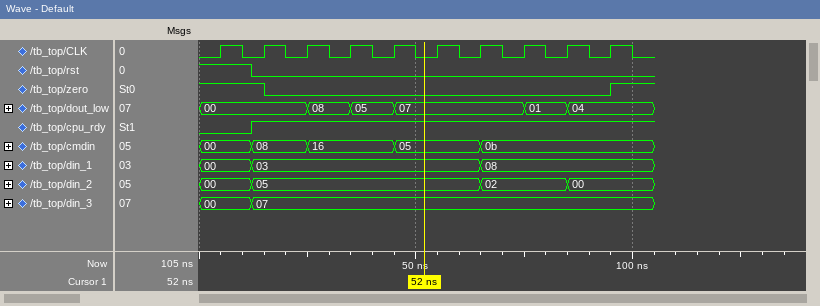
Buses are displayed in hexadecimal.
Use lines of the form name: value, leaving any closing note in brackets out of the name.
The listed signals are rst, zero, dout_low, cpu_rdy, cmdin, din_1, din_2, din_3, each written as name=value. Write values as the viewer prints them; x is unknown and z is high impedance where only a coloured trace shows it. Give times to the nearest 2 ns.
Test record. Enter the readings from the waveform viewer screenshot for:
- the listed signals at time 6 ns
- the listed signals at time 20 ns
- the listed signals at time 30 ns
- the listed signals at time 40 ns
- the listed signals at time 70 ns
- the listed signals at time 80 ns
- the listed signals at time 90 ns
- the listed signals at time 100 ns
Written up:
the listed signals at time 6 ns: rst=1, zero=1, dout_low=00, cpu_rdy=0, cmdin=00, din_1=00, din_2=00, din_3=00
the listed signals at time 20 ns: rst=0, zero=0, dout_low=00, cpu_rdy=1, cmdin=08, din_1=03, din_2=05, din_3=07
the listed signals at time 30 ns: rst=0, zero=0, dout_low=08, cpu_rdy=1, cmdin=16, din_1=03, din_2=05, din_3=07
the listed signals at time 40 ns: rst=0, zero=0, dout_low=05, cpu_rdy=1, cmdin=16, din_1=03, din_2=05, din_3=07
the listed signals at time 70 ns: rst=0, zero=0, dout_low=07, cpu_rdy=1, cmdin=0b, din_1=08, din_2=02, din_3=07
the listed signals at time 80 ns: rst=0, zero=0, dout_low=01, cpu_rdy=1, cmdin=0b, din_1=08, din_2=02, din_3=07
the listed signals at time 90 ns: rst=0, zero=0, dout_low=04, cpu_rdy=1, cmdin=0b, din_1=08, din_2=00, din_3=07
the listed signals at time 100 ns: rst=0, zero=1, dout_low=04, cpu_rdy=1, cmdin=0b, din_1=08, din_2=00, din_3=07
